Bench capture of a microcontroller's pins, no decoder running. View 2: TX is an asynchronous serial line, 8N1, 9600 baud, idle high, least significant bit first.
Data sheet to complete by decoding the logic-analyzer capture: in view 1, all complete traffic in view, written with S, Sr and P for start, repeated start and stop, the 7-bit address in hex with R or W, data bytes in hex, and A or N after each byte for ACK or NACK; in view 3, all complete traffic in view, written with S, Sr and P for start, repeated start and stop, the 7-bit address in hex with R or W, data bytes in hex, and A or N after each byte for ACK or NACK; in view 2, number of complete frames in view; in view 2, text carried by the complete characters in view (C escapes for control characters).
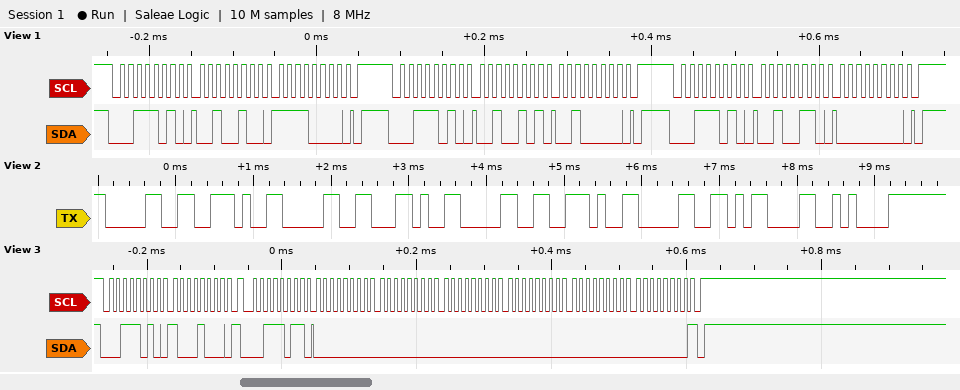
S 1DW A 24 A F0 A P S 1DW A 25 A 20 A P S 1DW A 26 A 00 A P
S 1DW A 88 A Sr 1DR A 00 A 00 A 00 A 00 A 00 A 00 N P
9
"0.0,0.0\r\n"
